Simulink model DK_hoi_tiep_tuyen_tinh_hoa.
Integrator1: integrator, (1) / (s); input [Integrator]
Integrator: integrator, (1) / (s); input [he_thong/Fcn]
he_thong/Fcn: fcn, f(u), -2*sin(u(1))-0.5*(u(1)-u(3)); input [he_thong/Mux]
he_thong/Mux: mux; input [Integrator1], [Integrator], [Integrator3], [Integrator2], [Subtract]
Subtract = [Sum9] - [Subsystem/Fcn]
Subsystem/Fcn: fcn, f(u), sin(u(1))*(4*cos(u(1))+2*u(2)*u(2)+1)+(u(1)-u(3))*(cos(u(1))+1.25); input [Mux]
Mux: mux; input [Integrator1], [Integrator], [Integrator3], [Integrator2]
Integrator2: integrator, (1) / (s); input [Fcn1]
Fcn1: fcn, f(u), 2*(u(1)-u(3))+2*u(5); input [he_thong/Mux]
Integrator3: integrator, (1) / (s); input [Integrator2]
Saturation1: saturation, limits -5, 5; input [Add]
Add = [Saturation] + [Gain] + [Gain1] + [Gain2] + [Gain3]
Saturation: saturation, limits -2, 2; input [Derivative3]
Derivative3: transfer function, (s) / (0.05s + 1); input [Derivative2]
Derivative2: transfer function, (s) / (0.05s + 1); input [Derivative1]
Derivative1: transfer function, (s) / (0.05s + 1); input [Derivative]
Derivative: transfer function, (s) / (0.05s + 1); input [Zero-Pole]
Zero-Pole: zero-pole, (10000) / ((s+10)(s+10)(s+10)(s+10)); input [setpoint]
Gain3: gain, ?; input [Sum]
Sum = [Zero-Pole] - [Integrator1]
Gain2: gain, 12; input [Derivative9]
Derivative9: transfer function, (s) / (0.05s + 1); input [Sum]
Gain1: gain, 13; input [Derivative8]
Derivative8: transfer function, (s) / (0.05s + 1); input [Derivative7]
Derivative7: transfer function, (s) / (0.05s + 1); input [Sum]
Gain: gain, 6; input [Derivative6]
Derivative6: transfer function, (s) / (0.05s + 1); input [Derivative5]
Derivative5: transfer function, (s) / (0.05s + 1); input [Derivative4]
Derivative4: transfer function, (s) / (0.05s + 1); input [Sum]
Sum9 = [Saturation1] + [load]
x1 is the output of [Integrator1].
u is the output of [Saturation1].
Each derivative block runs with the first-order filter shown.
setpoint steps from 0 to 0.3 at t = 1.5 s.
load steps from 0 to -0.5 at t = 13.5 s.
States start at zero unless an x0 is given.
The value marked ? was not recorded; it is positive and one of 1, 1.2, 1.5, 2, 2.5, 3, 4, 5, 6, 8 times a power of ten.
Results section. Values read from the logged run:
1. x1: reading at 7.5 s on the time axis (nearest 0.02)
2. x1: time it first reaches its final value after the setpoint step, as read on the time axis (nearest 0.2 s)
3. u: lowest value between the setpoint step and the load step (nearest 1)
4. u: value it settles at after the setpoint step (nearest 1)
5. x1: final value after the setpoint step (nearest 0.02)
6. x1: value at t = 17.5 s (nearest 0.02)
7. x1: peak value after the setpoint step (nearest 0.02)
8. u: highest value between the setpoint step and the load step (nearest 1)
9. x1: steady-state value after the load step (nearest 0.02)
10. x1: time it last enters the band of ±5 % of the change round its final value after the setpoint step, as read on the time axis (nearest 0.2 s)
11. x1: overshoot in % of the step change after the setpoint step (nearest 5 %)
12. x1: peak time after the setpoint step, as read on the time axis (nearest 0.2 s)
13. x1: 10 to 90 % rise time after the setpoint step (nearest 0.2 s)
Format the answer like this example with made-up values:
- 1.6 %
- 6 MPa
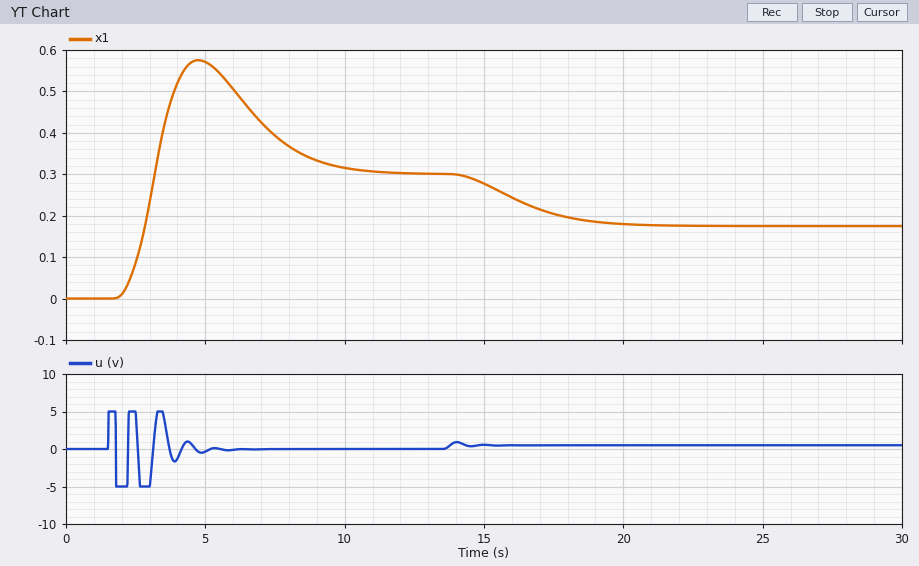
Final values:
- 0.40
- 3.2 s
- -5
- 0
- 0.30
- 0.20
- 0.58
- 5
- 0.18
- 10.0 s
- 90 %
- 4.8 s
- 1.0 s
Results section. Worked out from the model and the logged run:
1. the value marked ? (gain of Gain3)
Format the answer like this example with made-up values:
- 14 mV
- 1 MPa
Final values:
- 4
